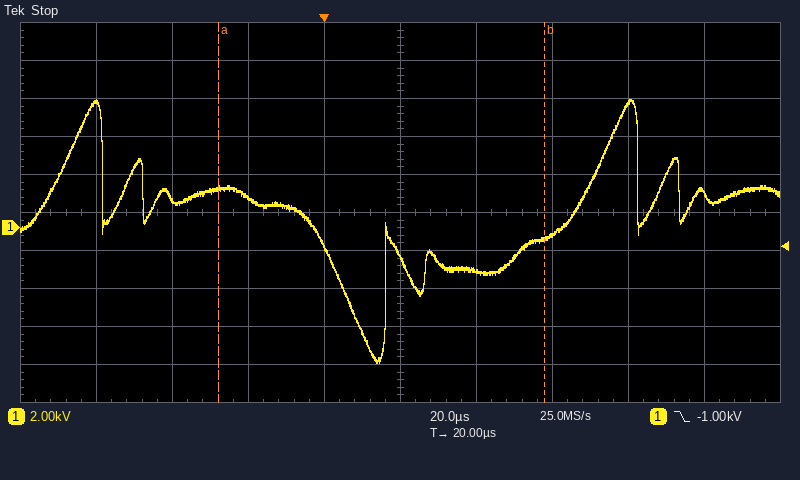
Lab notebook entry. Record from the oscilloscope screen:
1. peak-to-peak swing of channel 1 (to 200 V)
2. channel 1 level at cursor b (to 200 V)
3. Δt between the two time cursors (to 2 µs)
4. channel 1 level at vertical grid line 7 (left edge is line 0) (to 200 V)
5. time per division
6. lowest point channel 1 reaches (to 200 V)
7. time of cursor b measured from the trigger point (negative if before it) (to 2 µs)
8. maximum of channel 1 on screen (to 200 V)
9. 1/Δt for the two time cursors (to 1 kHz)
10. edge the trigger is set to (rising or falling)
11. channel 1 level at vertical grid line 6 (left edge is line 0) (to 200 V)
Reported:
13.8 kV
-600 V
86 µs
-400 V
20 µs
-7.0 kV
+58 µs
6.8 kV
12 kHz
falling
-2.2 kV
